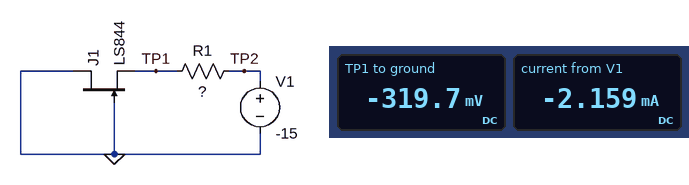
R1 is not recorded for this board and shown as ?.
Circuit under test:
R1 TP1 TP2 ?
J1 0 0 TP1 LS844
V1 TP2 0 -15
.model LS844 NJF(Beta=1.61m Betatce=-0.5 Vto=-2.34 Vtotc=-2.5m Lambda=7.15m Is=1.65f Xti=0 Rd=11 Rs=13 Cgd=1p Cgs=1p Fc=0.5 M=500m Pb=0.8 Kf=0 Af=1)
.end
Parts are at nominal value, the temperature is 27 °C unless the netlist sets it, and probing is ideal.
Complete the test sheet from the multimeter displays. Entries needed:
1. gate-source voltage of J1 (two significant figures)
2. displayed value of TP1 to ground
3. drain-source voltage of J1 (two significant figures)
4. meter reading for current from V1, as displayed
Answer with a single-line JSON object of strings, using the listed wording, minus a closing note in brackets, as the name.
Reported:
{"gate-source voltage of J1": "320 mV", "displayed value of TP1 to ground": "-319.7 mV", "drain-source voltage of J1": "320 mV", "meter reading for current from V1, as displayed": "-2.159 mA"}
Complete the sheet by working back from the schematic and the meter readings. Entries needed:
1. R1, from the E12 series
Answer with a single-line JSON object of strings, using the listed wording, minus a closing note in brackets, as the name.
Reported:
{"R1, from the E12 series": "6.8 kΩ"}
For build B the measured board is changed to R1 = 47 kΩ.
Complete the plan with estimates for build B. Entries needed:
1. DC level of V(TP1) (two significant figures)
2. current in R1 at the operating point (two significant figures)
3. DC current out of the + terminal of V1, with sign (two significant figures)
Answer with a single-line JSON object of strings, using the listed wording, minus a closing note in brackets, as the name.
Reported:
{"DC level of V(TP1)": "-49 mV", "current in R1 at the operating point": "320 µA", "DC current out of the + terminal of V1, with sign": "-320 µA"}
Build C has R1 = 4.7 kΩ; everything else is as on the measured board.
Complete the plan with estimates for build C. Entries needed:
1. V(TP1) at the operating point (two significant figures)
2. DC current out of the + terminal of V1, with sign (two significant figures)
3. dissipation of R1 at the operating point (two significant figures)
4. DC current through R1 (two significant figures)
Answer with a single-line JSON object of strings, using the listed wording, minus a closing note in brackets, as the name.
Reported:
{"V(TP1) at the operating point": "-450 mV", "DC current out of the + terminal of V1, with sign": "-3.1 mA", "dissipation of R1 at the operating point": "45 mW", "DC current through R1": "3.1 mA"}
